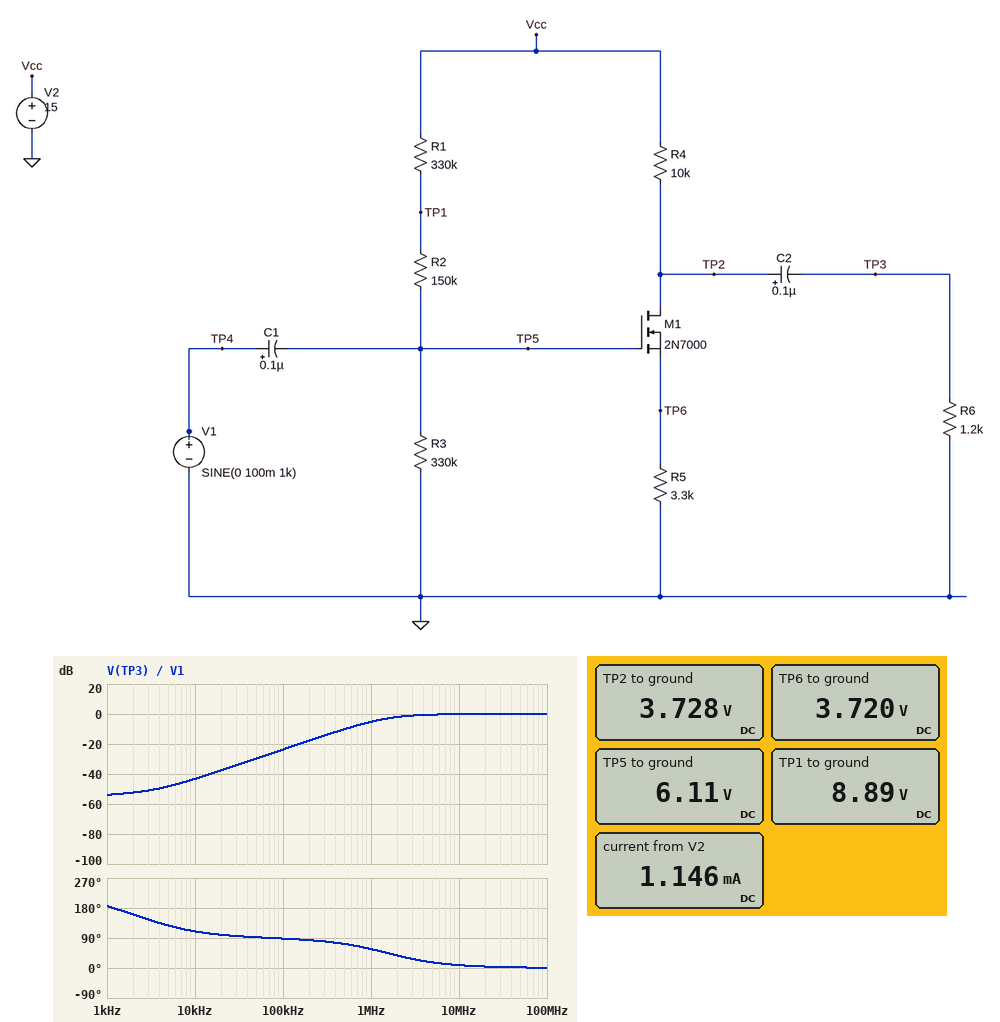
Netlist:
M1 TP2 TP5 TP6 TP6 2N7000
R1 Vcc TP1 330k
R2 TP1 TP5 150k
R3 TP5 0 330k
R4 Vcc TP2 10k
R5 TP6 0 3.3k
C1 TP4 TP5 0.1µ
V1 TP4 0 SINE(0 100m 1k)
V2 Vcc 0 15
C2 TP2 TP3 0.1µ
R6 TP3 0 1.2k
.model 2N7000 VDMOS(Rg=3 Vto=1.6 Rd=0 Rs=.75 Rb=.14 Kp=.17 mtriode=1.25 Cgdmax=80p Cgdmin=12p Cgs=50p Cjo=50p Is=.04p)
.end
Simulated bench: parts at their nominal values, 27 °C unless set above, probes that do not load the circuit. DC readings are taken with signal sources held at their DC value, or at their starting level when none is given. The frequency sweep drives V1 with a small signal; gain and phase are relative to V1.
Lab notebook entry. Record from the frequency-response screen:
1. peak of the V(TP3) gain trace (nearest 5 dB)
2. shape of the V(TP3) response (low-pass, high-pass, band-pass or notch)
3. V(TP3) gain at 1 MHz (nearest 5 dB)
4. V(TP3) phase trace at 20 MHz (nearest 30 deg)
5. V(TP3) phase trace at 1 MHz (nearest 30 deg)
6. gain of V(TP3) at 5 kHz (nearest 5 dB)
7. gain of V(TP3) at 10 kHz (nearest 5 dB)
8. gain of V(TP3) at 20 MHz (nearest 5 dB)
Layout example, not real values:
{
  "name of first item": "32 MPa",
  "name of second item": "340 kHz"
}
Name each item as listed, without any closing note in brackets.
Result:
{
  "peak of the V(TP3) gain trace": "0 dB",
  "shape of the V(TP3) response": "high-pass",
  "V(TP3) gain at 1 MHz": "-5 dB",
  "V(TP3) phase trace at 20 MHz": "0 deg",
  "V(TP3) phase trace at 1 MHz": "60 deg",
  "gain of V(TP3) at 5 kHz": "-50 dB",
  "gain of V(TP3) at 10 kHz": "-45 dB",
  "gain of V(TP3) at 20 MHz": "0 dB"
}
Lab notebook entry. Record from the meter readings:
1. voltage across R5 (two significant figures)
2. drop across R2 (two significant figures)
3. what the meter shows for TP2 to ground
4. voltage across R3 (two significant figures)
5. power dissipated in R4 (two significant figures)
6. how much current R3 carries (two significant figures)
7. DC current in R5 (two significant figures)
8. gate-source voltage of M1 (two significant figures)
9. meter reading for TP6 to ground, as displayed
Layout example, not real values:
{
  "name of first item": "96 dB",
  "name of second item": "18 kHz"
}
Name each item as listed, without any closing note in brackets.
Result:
{
  "voltage across R5": "3.7 V",
  "drop across R2": "2.8 V",
  "what the meter shows for TP2 to ground": "3.728 V",
  "voltage across R3": "6.1 V",
  "power dissipated in R4": "13 mW",
  "how much current R3 carries": "19 µA",
  "DC current in R5": "1.1 mA",
  "gate-source voltage of M1": "2.4 V",
  "meter reading for TP6 to ground, as displayed": "3.720 V"
}
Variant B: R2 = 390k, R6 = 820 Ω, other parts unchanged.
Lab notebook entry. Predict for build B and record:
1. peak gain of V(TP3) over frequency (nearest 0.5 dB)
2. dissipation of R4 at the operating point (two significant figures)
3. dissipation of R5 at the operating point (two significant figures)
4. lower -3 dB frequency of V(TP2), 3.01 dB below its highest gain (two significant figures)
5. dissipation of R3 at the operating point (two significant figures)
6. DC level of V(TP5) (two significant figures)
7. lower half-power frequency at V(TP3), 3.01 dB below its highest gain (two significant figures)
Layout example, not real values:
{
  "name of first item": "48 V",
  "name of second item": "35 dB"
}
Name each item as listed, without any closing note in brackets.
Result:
{
  "peak gain of V(TP3) over frequency": "0.5 dB",
  "dissipation of R4 at the operating point": "8.6 mW",
  "dissipation of R5 at the operating point": "2.8 mW",
  "lower -3 dB frequency of V(TP2), 3.01 dB below its highest gain": "6.4 Hz",
  "dissipation of R3 at the operating point": "67 µW",
  "DC level of V(TP5)": "4.7 V",
  "lower half-power frequency at V(TP3), 3.01 dB below its highest gain": "5.3 MHz"
}
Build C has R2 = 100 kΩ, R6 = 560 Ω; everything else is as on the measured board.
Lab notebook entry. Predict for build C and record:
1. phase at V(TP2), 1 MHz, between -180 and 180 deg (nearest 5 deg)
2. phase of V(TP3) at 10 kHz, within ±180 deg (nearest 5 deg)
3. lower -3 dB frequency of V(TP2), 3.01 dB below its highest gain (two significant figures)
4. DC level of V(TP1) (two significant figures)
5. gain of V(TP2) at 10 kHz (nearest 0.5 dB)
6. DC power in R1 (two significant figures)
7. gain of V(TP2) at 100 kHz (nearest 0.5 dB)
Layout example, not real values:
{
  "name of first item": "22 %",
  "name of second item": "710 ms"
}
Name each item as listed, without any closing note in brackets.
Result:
{
  "phase at V(TP2), 1 MHz, between -180 and 180 deg": "70 deg",
  "phase of V(TP3) at 10 kHz, within ±180 deg": "100 deg",
  "lower -3 dB frequency of V(TP2), 3.01 dB below its highest gain": "2.7 MHz",
  "DC level of V(TP1)": "8.5 V",
  "gain of V(TP2) at 10 kHz": "-48.0 dB",
  "DC power in R1": "130 µW",
  "gain of V(TP2) at 100 kHz": "-28.5 dB"
}
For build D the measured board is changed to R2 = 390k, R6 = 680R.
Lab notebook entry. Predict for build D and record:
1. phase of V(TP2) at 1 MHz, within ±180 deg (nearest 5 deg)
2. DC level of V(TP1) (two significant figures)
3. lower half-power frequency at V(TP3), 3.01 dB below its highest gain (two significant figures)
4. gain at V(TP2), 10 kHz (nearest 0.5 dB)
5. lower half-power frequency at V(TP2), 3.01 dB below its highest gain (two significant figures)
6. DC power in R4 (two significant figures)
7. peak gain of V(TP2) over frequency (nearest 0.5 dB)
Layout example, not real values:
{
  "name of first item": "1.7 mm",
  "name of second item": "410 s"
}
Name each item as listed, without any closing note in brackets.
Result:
{
  "phase of V(TP2) at 1 MHz, within ±180 deg": "135 deg",
  "DC level of V(TP1)": "10 V",
  "lower half-power frequency at V(TP3), 3.01 dB below its highest gain": "6.2 MHz",
  "gain at V(TP2), 10 kHz": "-14.5 dB",
  "lower half-power frequency at V(TP2), 3.01 dB below its highest gain": "6.4 Hz",
  "DC power in R4": "8.6 mW",
  "peak gain of V(TP2) over frequency": "9.0 dB"
}
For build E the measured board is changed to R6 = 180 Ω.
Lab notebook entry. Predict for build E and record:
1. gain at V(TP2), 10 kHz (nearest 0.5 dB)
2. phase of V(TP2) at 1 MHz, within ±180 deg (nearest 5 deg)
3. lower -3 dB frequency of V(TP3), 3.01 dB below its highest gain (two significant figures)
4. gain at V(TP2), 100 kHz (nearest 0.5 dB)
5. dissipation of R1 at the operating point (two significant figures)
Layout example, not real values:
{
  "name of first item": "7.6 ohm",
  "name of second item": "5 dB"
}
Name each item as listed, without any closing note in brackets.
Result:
{
  "gain at V(TP2), 10 kHz": "-54.5 dB",
  "phase of V(TP2) at 1 MHz, within ±180 deg": "80 deg",
  "lower -3 dB frequency of V(TP3), 3.01 dB below its highest gain": "7.3 MHz",
  "gain at V(TP2), 100 kHz": "-37.5 dB",
  "dissipation of R1 at the operating point": "110 µW"
}
